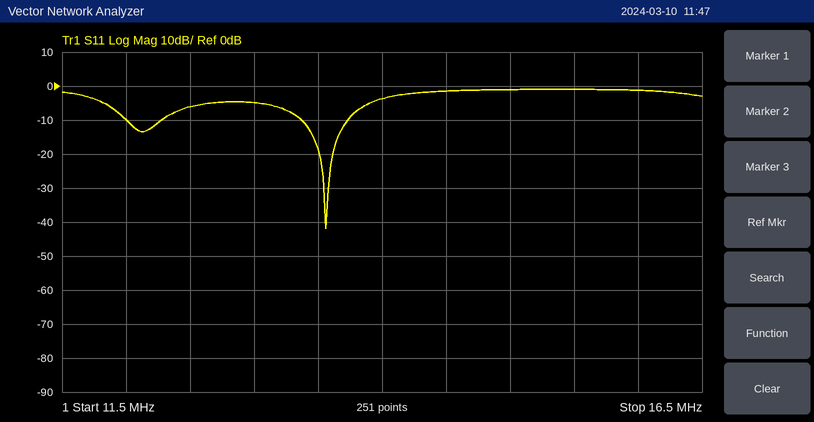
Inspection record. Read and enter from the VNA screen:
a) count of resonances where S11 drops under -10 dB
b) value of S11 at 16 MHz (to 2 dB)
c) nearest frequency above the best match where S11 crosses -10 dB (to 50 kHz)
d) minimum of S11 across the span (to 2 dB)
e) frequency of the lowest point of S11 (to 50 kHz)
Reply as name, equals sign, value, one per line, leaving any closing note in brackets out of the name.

count of resonances where S11 drops under -10 dB = 2
value of S11 at 16 MHz = -2 dB
nearest frequency above the best match where S11 crosses -10 dB = 13.75 MHz
minimum of S11 across the span = -42 dB
frequency of the lowest point of S11 = 13.55 MHz
